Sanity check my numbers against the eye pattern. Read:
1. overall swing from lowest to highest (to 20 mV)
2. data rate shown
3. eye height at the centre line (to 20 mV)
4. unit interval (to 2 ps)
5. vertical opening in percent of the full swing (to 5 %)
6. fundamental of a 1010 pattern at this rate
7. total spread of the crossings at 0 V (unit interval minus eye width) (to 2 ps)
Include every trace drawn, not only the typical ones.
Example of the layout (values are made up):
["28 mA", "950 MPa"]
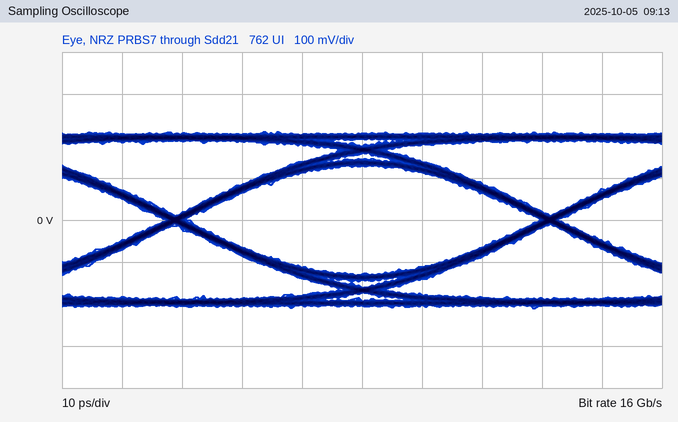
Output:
["420 mV", "16 Gb/s", "260 mV", "62 ps", "60 %", "8 GHz", "4 ps"]
